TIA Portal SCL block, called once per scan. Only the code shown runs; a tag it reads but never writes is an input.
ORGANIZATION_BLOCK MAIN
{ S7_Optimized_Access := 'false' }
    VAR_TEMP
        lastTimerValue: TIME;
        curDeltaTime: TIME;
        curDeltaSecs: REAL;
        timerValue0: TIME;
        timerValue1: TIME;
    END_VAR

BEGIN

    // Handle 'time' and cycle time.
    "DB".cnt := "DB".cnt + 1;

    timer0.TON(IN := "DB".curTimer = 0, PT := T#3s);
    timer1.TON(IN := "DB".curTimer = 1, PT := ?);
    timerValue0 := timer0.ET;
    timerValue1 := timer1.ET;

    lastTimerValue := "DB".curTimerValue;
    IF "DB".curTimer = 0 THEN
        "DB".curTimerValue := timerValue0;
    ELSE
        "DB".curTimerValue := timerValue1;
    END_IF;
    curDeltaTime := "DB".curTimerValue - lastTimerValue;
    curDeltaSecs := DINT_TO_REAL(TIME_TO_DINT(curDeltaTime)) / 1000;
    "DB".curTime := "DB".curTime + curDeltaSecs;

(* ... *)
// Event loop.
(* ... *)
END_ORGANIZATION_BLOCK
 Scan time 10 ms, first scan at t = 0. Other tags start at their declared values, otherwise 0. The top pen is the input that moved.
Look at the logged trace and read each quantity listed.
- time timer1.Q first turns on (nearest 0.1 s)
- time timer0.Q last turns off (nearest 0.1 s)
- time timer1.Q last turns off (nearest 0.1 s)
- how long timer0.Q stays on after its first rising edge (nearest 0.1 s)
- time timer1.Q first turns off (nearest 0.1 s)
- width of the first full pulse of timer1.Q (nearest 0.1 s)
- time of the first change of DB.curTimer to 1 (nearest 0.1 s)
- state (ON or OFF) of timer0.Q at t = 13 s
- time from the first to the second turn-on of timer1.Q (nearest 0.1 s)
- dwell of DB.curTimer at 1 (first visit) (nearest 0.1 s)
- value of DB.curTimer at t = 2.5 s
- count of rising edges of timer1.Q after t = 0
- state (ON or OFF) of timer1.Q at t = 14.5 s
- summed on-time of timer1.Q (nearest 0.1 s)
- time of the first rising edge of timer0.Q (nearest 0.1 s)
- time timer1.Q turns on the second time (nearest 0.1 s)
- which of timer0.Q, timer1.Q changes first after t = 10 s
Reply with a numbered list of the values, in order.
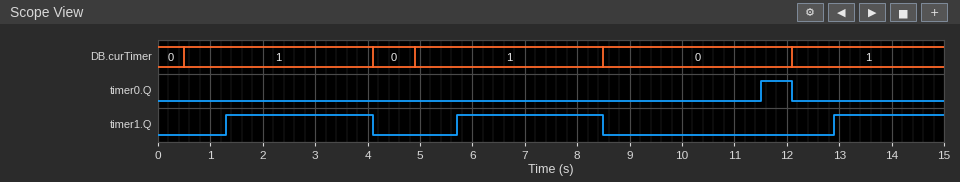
1. 1.3 s
2. 12.1 s
3. 8.5 s
4. 0.6 s
5. 4.1 s
6. 2.8 s
7. 0.5 s
8. OFF
9. 4.4 s
10. 3.6 s
11. 1
12. 3
13. ON
14. 7.7 s
15. 11.5 s
16. 5.7 s
17. timer0.Q
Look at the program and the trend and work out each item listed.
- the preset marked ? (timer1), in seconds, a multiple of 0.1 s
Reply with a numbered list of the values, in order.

1. 0.8 s
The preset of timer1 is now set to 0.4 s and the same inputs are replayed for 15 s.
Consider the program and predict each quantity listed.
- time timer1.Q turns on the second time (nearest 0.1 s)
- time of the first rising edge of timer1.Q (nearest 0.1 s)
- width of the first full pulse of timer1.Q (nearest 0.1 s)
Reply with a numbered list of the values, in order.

1. 5.3 s
2. 0.9 s
3. 3.2 s
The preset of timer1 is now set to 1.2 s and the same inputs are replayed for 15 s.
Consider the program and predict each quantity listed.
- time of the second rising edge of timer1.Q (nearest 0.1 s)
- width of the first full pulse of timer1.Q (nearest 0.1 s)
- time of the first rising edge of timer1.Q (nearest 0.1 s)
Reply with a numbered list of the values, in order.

1. 6.1 s
2. 2.4 s
3. 1.7 s
